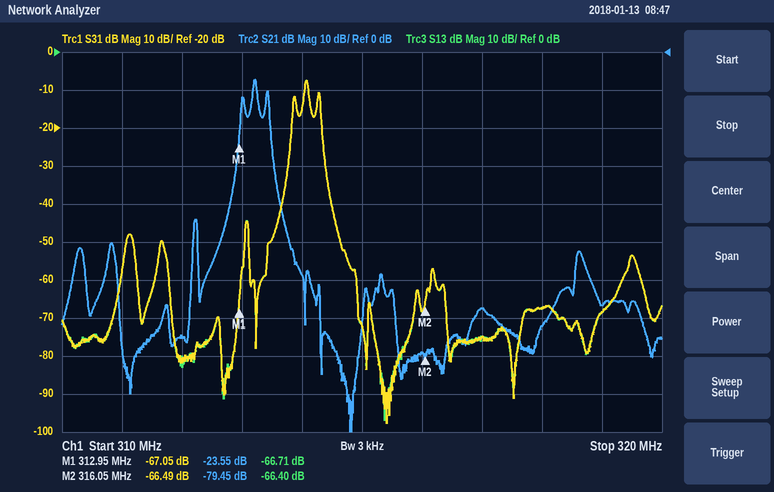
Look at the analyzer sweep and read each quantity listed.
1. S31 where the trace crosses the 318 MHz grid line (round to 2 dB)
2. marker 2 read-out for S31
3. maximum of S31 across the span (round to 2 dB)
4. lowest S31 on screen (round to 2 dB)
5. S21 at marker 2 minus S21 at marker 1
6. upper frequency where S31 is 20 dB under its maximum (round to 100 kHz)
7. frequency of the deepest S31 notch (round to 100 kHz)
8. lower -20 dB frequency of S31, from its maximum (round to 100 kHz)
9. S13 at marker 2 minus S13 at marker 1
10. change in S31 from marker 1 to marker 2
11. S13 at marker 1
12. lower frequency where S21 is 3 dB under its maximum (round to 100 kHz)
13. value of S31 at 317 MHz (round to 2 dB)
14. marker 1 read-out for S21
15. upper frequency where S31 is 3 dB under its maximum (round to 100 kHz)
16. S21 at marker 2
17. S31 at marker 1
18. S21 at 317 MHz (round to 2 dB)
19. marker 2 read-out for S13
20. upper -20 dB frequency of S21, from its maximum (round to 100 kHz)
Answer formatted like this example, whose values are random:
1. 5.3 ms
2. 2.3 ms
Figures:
1. -68 dB
2. -66.49 dB
3. -8 dB
4. -98 dB
5. -55.90 dB
6. 314.4 MHz
7. 315.4 MHz
8. 313.8 MHz
9. 0.31 dB
10. 0.56 dB
11. -66.71 dB
12. 313.2 MHz
13. -76 dB
14. -23.55 dB
15. 314.1 MHz
16. -79.45 dB
17. -67.05 dB
18. -68 dB
19. -66.40 dB
20. 313.5 MHz
